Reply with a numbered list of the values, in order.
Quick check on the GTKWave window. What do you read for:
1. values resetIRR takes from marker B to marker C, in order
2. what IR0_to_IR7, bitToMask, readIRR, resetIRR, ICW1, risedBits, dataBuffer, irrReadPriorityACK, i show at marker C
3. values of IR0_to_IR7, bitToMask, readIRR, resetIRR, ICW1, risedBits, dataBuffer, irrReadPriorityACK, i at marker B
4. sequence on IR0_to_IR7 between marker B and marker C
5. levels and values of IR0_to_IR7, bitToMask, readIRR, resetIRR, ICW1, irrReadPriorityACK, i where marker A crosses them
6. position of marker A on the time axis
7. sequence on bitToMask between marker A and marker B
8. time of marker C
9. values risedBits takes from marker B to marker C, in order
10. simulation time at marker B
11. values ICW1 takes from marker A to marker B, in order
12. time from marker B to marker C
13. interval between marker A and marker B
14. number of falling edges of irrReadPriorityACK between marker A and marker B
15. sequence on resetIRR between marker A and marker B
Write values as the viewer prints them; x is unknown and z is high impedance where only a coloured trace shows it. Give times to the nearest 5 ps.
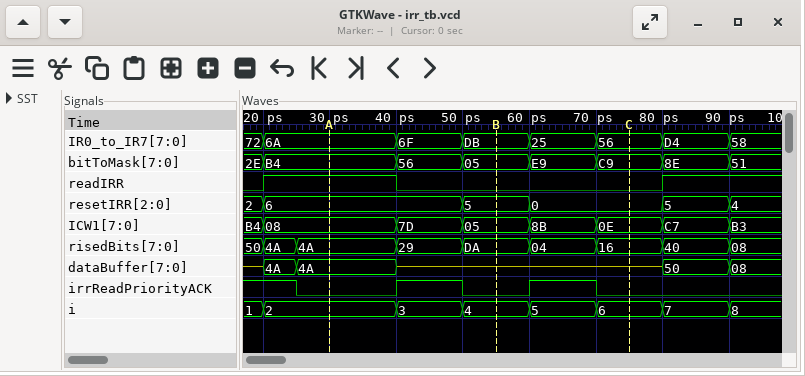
1. 5, 0
2. IR0_to_IR7=56, bitToMask=C9, readIRR=0, resetIRR=0, ICW1=0E, risedBits=16, dataBuffer=z, irrReadPriorityACK=0, i=6
3. IR0_to_IR7=DB, bitToMask=05, readIRR=0, resetIRR=5, ICW1=05, risedBits=DA, dataBuffer=z, irrReadPriorityACK=0, i=4
4. DB, 25, 56
5. IR0_to_IR7=6A, bitToMask=B4, readIRR=1, resetIRR=6, ICW1=08, irrReadPriorityACK=0, i=2
6. 30 ps
7. B4, 56, 05
8. 75 ps
9. DA, 04, 16
10. 55 ps
11. 08, 7D, 05
12. 20 ps
13. 25 ps
14. 1
15. 6, 5
